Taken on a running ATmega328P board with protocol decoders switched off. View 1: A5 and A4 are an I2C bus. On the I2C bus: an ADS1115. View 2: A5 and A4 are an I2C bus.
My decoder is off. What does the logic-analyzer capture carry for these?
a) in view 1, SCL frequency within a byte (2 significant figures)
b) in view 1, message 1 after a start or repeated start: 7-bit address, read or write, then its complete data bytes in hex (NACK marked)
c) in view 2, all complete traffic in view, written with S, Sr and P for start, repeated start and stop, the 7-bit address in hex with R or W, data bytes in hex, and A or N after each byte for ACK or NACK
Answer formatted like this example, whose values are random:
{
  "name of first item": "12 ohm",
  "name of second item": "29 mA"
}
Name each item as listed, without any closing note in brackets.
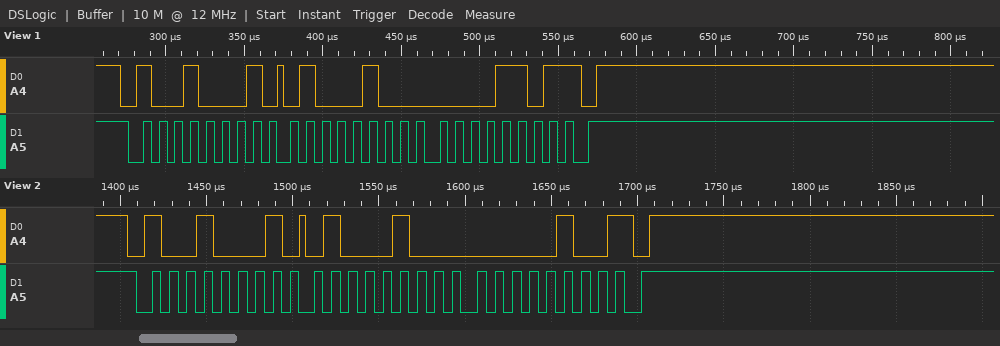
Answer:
{
  "in view 1, SCL frequency within a byte": "100 kHz",
  "in view 1, message 1 after a start or repeated start: 7-bit address, read or write, then its complete data bytes in hex": "0x48 read: 44 0D NACK",
  "in view 2, all complete traffic in view, written with S, Sr and P for start, repeated start and stop, the 7-bit address in hex with R or W, data bytes in hex, and A or N after each byte for ACK or NACK": "S 48R A 44 A 04 N P"
}
